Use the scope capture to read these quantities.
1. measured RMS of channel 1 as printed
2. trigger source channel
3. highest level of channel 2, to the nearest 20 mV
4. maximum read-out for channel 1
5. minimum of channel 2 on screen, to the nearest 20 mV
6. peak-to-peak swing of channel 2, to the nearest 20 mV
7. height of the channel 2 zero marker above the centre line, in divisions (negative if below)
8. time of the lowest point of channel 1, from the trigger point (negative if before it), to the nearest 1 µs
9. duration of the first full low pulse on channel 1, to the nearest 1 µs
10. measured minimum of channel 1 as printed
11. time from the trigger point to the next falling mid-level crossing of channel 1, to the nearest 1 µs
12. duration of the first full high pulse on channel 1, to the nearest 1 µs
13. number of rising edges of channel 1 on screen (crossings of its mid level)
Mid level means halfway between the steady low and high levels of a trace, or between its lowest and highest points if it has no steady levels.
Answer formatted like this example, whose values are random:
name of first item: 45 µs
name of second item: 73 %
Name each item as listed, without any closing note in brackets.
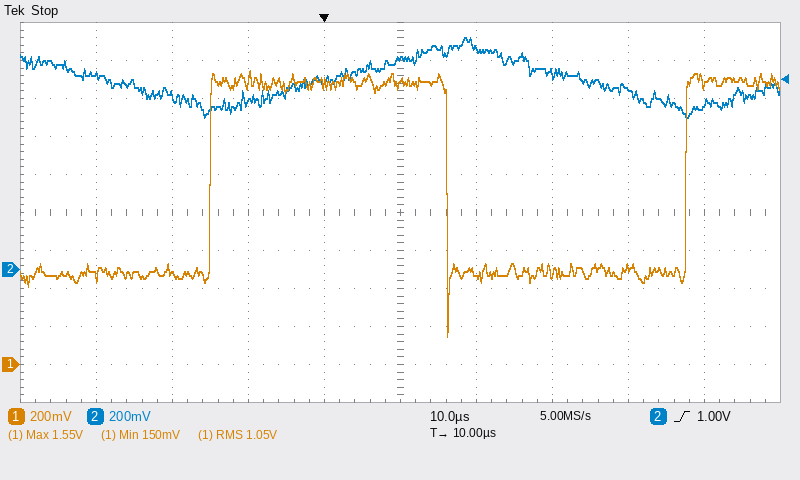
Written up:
measured RMS of channel 1 as printed: 1.05 V
trigger source channel: channel 2
highest level of channel 2, to the nearest 20 mV: 1.22 V
maximum read-out for channel 1: 1.55 V
minimum of channel 2 on screen, to the nearest 20 mV: 800 mV
peak-to-peak swing of channel 2, to the nearest 20 mV: 420 mV
height of the channel 2 zero marker above the centre line, in divisions: -1.5 div
time of the lowest point of channel 1, from the trigger point (negative if before it), to the nearest 1 µs: +16 µs
duration of the first full low pulse on channel 1, to the nearest 1 µs: 31 µs
measured minimum of channel 1 as printed: 150 mV
time from the trigger point to the next falling mid-level crossing of channel 1, to the nearest 1 µs: 16 µs
duration of the first full high pulse on channel 1, to the nearest 1 µs: 31 µs
number of rising edges of channel 1 on screen: 2
